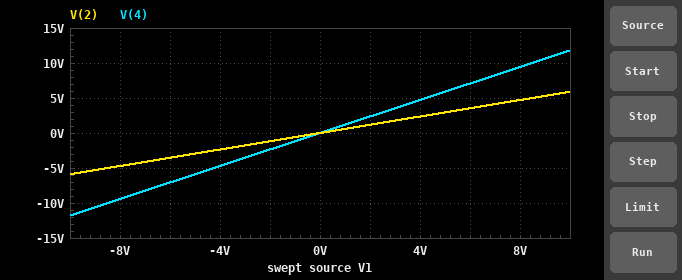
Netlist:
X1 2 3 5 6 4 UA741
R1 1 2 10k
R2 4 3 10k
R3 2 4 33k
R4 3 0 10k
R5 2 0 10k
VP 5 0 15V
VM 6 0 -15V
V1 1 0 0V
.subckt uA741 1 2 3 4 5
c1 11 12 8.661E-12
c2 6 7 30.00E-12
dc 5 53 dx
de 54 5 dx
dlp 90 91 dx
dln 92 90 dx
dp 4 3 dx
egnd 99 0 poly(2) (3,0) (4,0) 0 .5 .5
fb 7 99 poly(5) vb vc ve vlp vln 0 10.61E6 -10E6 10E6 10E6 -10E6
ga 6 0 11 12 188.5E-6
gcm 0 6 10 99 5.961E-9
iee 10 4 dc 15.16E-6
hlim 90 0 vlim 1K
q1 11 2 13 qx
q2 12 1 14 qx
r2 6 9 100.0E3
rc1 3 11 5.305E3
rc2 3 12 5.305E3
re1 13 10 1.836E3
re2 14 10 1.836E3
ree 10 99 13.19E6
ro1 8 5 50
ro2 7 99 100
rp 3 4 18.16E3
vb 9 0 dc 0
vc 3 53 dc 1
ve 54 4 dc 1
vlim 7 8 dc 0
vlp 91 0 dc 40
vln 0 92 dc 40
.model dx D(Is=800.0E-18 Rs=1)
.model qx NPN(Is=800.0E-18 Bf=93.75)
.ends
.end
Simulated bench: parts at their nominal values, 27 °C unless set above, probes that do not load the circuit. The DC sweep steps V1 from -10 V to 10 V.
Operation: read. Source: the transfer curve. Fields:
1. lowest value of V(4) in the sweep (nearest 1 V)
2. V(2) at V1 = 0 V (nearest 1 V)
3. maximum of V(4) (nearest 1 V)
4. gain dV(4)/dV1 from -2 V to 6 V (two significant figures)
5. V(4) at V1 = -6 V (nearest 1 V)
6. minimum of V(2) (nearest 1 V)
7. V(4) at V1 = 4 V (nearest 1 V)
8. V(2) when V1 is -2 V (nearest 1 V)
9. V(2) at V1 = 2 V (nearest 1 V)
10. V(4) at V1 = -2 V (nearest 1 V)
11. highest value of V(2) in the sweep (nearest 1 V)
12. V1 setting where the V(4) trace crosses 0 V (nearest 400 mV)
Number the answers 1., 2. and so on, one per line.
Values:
1. -12 V
2. 0 V
3. 12 V
4. 1.2 V/V
5. -7 V
6. -6 V
7. 5 V
8. -1 V
9. 1 V
10. -2 V
11. 6 V
12. 0 V
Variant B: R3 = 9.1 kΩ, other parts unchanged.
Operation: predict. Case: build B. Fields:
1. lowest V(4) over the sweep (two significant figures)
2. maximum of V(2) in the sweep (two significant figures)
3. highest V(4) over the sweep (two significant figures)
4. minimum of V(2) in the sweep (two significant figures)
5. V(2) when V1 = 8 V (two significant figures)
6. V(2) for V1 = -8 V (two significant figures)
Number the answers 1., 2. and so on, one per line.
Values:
1. -15 V
2. 8.4 V
3. 15 V
4. -8.4 V
5. 7.8 V
6. -7.8 V
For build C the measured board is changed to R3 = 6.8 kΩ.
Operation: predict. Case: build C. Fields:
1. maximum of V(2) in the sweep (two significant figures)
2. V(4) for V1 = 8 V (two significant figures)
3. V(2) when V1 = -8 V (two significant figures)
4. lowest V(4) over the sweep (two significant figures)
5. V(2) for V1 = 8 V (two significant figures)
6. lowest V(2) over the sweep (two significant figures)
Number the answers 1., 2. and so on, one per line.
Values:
1. 9.1 V
2. 15 V
3. -8.5 V
4. -15 V
5. 8.5 V
6. -9.1 V
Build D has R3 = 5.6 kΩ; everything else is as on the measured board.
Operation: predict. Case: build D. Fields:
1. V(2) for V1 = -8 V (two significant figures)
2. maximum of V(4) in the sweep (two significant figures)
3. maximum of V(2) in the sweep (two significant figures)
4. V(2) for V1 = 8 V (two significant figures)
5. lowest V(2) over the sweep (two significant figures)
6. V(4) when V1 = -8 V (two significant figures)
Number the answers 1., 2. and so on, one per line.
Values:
1. -9.0 V
2. 15 V
3. 9.5 V
4. 9.0 V
5. -9.5 V
6. -15 V
